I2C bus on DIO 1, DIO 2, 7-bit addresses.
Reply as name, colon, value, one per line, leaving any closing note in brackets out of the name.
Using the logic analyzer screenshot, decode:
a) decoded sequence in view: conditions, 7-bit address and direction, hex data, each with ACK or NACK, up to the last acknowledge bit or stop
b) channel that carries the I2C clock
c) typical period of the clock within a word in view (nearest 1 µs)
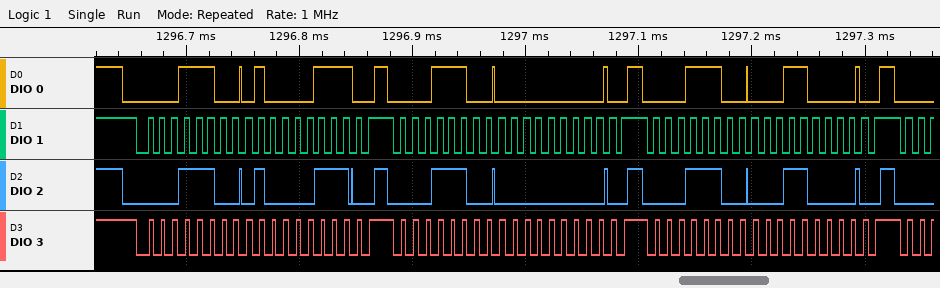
decoded sequence in view: conditions, 7-bit address and direction, hex data, each with ACK or NACK, up to the last acknowledge bit or stop: start, address 0E write ACK, 87 ACK, stop, start, address 0E write ACK, 00 ACK, stop, start, address 0E write ACK, 30 ACK, stop
channel that carries the I2C clock: DIO 1
typical period of the clock within a word in view: 11 µs
